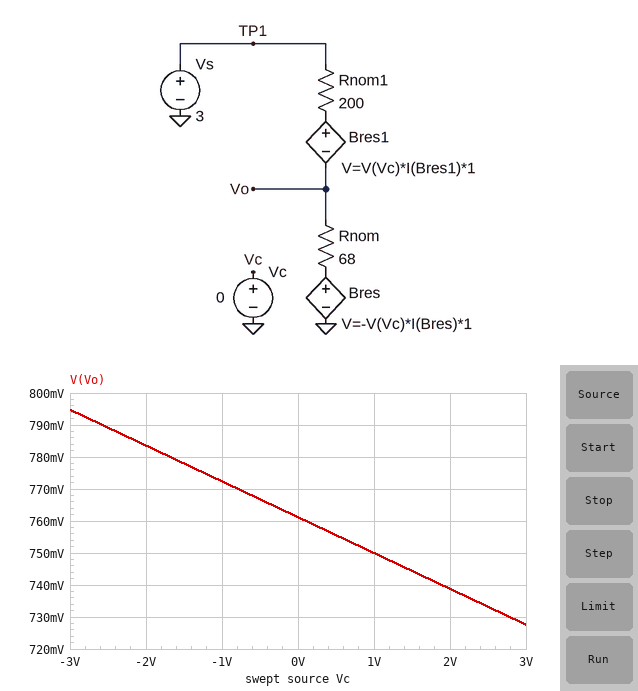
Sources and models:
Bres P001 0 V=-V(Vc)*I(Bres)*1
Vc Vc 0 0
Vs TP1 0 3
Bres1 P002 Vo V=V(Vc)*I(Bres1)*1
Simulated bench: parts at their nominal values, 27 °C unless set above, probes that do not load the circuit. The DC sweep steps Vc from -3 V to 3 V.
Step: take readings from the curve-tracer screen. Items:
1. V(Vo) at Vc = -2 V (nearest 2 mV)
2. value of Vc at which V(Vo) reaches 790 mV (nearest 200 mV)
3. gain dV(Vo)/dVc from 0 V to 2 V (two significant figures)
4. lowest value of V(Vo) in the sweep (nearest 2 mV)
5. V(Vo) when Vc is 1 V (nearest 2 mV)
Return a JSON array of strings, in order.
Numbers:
["784 mV", "-2.6 V", "-0.011 V/V", "728 mV", "750 mV"]
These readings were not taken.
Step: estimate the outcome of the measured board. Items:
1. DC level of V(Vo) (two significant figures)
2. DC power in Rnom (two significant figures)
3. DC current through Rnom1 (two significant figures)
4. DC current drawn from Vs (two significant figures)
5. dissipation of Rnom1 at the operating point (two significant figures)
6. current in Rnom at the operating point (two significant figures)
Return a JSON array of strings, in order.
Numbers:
["760 mV", "8.5 mW", "11 mA", "11 mA", "25 mW", "11 mA"]
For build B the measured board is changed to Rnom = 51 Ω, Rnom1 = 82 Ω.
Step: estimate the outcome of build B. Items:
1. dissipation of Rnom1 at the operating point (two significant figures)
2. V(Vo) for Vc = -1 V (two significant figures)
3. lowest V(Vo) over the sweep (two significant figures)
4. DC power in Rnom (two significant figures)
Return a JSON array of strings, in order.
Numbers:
["42 mW", "1.2 V", "1.1 V", "26 mW"]
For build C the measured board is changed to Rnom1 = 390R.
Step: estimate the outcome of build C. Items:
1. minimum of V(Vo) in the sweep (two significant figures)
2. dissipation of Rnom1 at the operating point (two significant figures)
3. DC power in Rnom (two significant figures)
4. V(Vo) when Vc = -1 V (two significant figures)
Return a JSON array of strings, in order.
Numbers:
["430 mV", "17 mW", "2.9 mW", "450 mV"]
